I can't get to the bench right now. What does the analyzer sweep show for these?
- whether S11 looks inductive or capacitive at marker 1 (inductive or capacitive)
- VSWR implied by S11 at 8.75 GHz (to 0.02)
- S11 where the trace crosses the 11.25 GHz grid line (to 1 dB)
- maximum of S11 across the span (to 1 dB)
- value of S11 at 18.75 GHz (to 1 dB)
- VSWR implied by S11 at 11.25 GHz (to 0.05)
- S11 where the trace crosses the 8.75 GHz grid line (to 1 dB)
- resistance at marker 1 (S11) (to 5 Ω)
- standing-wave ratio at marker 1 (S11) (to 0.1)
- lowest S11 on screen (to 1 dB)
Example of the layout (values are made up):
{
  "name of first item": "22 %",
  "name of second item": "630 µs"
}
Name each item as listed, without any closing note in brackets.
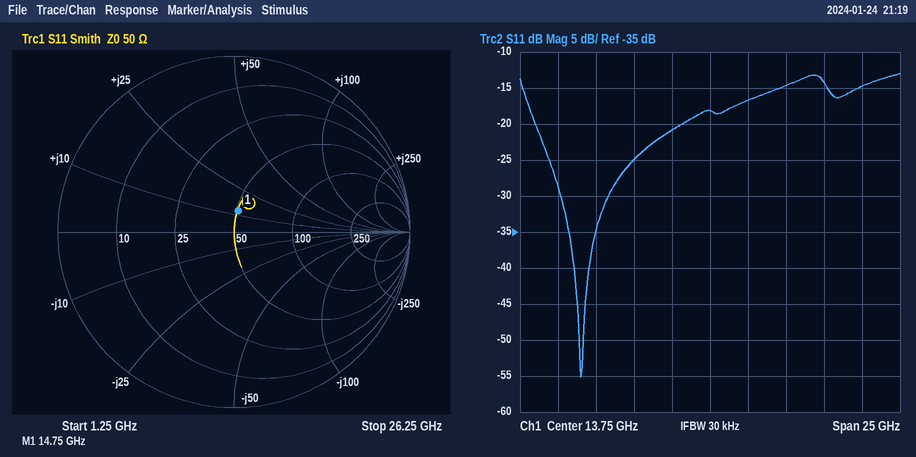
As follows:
{
  "whether S11 looks inductive or capacitive at marker 1": "inductive",
  "VSWR implied by S11 at 8.75 GHz": "1.12",
  "S11 where the trace crosses the 11.25 GHz grid line": "-21 dB",
  "maximum of S11 across the span": "-13 dB",
  "value of S11 at 18.75 GHz": "-15 dB",
  "VSWR implied by S11 at 11.25 GHz": "1.20",
  "S11 where the trace crosses the 8.75 GHz grid line": "-25 dB",
  "resistance at marker 1 (S11)": "50 Ω",
  "standing-wave ratio at marker 1 (S11)": "1.3",
  "lowest S11 on screen": "-55 dB"
}
